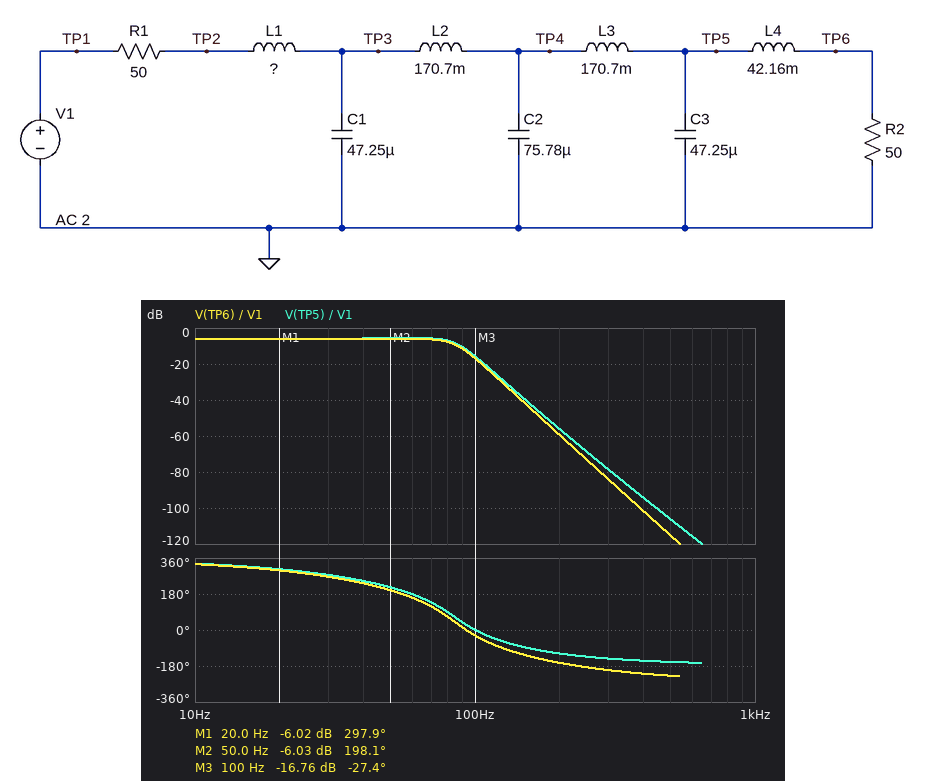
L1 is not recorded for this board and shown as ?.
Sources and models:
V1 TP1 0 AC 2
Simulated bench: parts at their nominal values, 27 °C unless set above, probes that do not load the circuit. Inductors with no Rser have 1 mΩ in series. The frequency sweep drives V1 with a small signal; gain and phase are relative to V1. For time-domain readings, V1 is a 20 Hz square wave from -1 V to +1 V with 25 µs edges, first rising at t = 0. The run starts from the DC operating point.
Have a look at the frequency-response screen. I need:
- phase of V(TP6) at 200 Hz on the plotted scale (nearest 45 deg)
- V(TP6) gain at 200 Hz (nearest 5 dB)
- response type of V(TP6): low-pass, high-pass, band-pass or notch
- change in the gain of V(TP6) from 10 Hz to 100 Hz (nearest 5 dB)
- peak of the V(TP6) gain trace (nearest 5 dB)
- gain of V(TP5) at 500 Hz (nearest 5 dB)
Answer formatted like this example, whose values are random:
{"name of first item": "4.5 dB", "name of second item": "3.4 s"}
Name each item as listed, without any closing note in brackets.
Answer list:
{"phase of V(TP6) at 200 Hz on the plotted scale": "-180 deg", "V(TP6) gain at 200 Hz": "-60 dB", "response type of V(TP6): low-pass, high-pass, band-pass or notch": "low-pass", "change in the gain of V(TP6) from 10 Hz to 100 Hz": "-10 dB", "peak of the V(TP6) gain trace": "-5 dB", "gain of V(TP5) at 500 Hz": "-105 dB"}
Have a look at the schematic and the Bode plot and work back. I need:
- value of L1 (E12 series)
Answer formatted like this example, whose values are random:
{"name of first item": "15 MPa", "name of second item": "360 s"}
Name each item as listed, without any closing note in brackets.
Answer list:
{"value of L1": "47 mH"}
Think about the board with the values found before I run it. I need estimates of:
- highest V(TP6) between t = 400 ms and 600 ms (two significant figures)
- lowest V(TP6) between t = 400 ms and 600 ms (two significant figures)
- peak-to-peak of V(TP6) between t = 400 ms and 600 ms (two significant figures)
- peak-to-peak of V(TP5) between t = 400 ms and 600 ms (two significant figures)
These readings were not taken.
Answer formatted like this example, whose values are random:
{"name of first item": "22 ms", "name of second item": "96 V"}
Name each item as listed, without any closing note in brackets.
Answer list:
{"highest V(TP6) between t = 400 ms and 600 ms": "650 mV", "lowest V(TP6) between t = 400 ms and 600 ms": "-650 mV", "peak-to-peak of V(TP6) between t = 400 ms and 600 ms": "1.3 V", "peak-to-peak of V(TP5) between t = 400 ms and 600 ms": "1.3 V"}
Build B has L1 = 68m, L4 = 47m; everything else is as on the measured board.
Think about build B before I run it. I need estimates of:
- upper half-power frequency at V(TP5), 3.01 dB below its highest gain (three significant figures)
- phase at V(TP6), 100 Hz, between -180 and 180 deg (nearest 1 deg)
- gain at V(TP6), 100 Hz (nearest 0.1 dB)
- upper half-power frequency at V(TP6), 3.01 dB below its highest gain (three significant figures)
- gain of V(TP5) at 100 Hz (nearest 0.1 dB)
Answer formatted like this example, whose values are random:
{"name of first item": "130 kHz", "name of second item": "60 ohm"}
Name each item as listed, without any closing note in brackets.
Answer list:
{"upper half-power frequency at V(TP5), 3.01 dB below its highest gain": "88.4 Hz", "phase at V(TP6), 100 Hz, between -180 and 180 deg": "-42 deg", "gain at V(TP6), 100 Hz": "-15.7 dB", "upper half-power frequency at V(TP6), 3.01 dB below its highest gain": "86.4 Hz", "gain of V(TP5) at 100 Hz": "-14.4 dB"}
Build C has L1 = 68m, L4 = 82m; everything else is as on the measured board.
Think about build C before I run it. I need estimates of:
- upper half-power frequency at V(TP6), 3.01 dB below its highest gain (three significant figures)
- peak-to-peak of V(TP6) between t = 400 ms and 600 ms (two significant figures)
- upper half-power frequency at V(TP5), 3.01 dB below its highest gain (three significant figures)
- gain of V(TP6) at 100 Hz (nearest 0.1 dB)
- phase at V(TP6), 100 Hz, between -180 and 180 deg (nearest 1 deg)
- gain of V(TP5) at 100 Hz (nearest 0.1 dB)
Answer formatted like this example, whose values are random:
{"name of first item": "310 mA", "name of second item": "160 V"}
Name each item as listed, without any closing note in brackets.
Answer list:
{"upper half-power frequency at V(TP6), 3.01 dB below its highest gain": "89.8 Hz", "peak-to-peak of V(TP6) between t = 400 ms and 600 ms": "1.3 V", "upper half-power frequency at V(TP5), 3.01 dB below its highest gain": "93.5 Hz", "gain of V(TP6) at 100 Hz": "-14.6 dB", "phase at V(TP6), 100 Hz, between -180 and 180 deg": "-64 deg", "gain of V(TP5) at 100 Hz": "-11.5 dB"}
